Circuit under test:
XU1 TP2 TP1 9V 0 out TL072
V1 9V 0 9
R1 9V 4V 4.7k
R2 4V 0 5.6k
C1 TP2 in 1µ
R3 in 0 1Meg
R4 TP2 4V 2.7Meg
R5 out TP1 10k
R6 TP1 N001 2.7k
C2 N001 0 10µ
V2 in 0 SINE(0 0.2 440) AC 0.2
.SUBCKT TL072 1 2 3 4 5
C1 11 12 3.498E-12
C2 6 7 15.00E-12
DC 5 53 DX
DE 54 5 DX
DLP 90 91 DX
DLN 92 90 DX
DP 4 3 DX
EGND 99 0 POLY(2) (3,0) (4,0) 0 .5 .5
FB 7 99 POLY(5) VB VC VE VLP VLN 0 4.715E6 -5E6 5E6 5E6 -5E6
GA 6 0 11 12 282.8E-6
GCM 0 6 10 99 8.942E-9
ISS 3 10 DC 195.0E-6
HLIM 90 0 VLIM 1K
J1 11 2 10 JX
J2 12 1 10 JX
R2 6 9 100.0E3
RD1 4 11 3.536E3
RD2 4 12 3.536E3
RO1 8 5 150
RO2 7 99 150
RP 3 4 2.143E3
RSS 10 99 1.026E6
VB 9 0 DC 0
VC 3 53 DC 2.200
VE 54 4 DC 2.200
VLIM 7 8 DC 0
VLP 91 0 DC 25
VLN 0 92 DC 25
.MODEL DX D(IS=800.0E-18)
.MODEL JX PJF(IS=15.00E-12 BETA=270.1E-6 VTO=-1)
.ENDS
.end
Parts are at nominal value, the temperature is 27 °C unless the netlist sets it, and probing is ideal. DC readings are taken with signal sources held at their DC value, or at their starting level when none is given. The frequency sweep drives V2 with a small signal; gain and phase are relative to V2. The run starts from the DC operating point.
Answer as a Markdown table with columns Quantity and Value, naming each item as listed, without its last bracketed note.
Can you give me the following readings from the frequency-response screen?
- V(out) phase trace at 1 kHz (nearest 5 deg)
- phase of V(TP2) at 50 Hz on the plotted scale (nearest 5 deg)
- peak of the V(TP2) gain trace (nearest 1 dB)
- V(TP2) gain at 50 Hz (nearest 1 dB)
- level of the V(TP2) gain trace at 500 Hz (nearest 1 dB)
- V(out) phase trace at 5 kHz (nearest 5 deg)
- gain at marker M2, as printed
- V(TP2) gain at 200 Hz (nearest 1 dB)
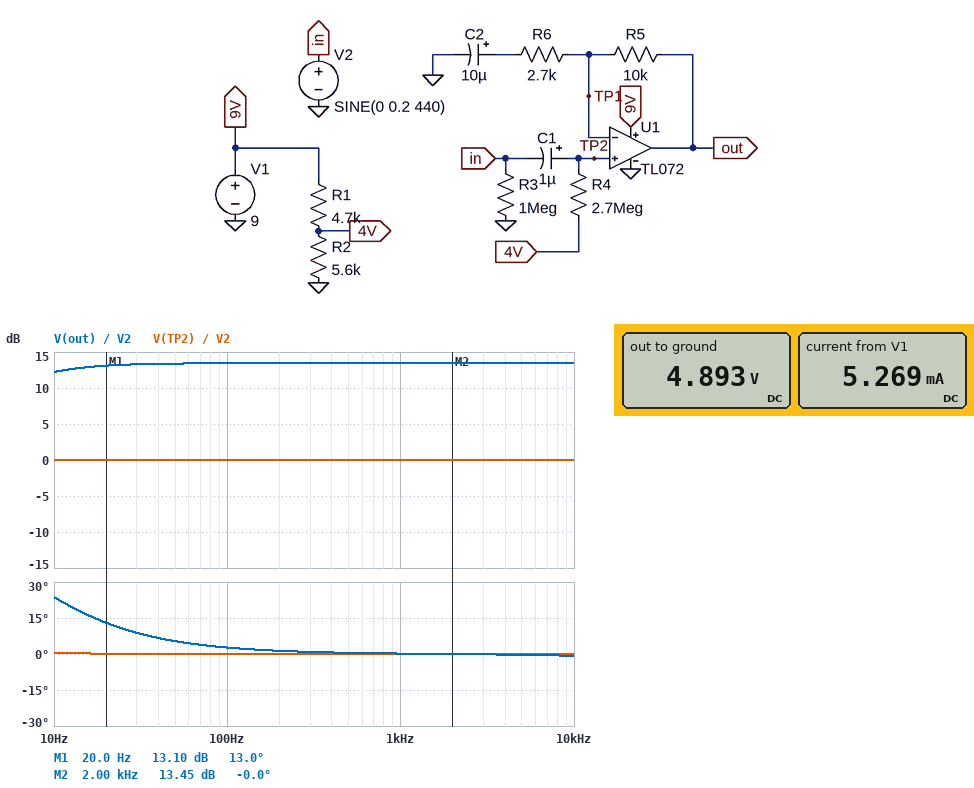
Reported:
| Quantity | Value |
|---|---|
| V(out) phase trace at 1 kHz | 0 deg |
| phase of V(TP2) at 50 Hz on the plotted scale | 0 deg |
| peak of the V(TP2) gain trace | 0 dB |
| V(TP2) gain at 50 Hz | 0 dB |
| level of the V(TP2) gain trace at 500 Hz | 0 dB |
| V(out) phase trace at 5 kHz | 0 deg |
| gain at marker M2, as printed | 13.45 dB |
| V(TP2) gain at 200 Hz | 0 dB |
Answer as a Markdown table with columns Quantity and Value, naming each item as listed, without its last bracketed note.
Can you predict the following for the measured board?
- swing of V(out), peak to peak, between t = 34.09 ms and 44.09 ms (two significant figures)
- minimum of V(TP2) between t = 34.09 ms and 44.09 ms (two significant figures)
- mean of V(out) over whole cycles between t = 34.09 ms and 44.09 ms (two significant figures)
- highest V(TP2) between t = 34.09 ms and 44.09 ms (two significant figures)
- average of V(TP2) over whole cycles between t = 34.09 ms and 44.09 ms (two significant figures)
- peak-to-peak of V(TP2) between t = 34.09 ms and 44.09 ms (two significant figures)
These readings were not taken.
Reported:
| Quantity | Value |
|---|---|
| swing of V(out), peak to peak, between t = 34.09 ms and 44.09 ms | 1.9 V |
| minimum of V(TP2) between t = 34.09 ms and 44.09 ms | 4.7 V |
| mean of V(out) over whole cycles between t = 34.09 ms and 44.09 ms | 4.9 V |
| highest V(TP2) between t = 34.09 ms and 44.09 ms | 5.1 V |
| average of V(TP2) over whole cycles between t = 34.09 ms and 44.09 ms | 4.9 V |
| peak-to-peak of V(TP2) between t = 34.09 ms and 44.09 ms | 400 mV |
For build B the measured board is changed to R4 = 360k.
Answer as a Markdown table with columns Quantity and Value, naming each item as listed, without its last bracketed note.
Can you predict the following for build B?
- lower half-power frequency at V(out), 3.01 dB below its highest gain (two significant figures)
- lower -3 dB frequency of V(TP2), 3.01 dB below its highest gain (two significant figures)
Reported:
| Quantity | Value |
|---|---|
| lower half-power frequency at V(out), 3.01 dB below its highest gain | 5.7 Hz |
| lower -3 dB frequency of V(TP2), 3.01 dB below its highest gain | 440 mHz |
